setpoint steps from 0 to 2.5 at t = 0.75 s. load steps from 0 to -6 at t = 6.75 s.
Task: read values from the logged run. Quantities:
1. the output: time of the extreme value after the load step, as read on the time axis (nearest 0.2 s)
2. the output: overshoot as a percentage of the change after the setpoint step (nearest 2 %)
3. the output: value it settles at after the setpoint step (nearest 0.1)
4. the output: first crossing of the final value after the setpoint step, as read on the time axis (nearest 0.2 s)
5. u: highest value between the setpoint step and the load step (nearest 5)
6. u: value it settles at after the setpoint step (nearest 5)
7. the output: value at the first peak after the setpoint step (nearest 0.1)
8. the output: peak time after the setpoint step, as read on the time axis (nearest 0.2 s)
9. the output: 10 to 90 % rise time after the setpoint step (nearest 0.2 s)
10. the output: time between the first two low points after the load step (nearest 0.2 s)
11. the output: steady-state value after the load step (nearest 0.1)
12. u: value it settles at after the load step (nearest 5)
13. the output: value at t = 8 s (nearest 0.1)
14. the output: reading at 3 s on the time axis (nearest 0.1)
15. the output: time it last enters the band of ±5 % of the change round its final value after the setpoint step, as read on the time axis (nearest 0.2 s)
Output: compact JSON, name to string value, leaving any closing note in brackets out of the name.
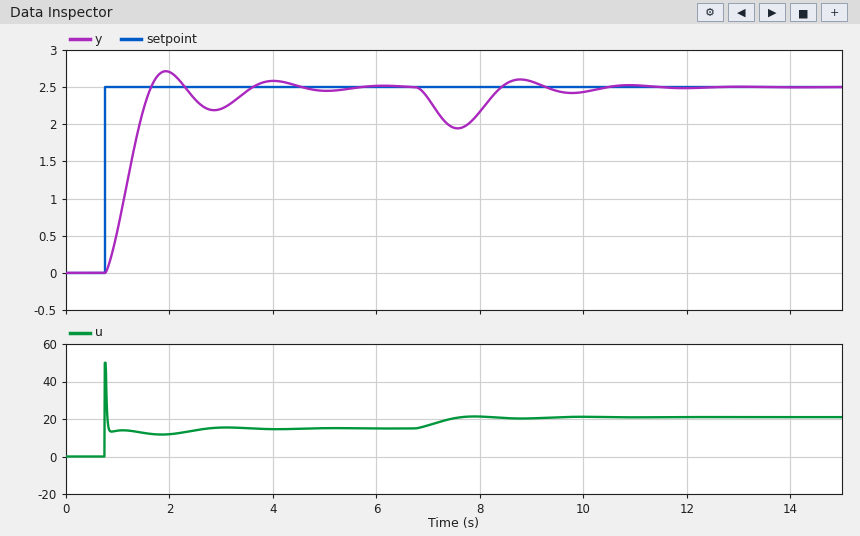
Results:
{"the output: time of the extreme value after the load step, as read on the time axis": "7.6 s", "the output: overshoot as a percentage of the change after the setpoint step": "8 %", "the output: value it settles at after the setpoint step": "2.5", "the output: first crossing of the final value after the setpoint step, as read on the time axis": "1.6 s", "u: highest value between the setpoint step and the load step": "50", "u: value it settles at after the setpoint step": "15", "the output: value at the first peak after the setpoint step": "2.7", "the output: peak time after the setpoint step, as read on the time axis": "2.0 s", "the output: 10 to 90 % rise time after the setpoint step": "0.6 s", "the output: time between the first two low points after the load step": "2.2 s", "the output: steady-state value after the load step": "2.5", "u: value it settles at after the load step": "20", "the output: value at t = 8 s": "2.2", "the output: reading at 3 s on the time axis": "2.2", "the output: time it last enters the band of ±5 % of the change round its final value after the setpoint step, as read on the time axis": "3.4 s"}
